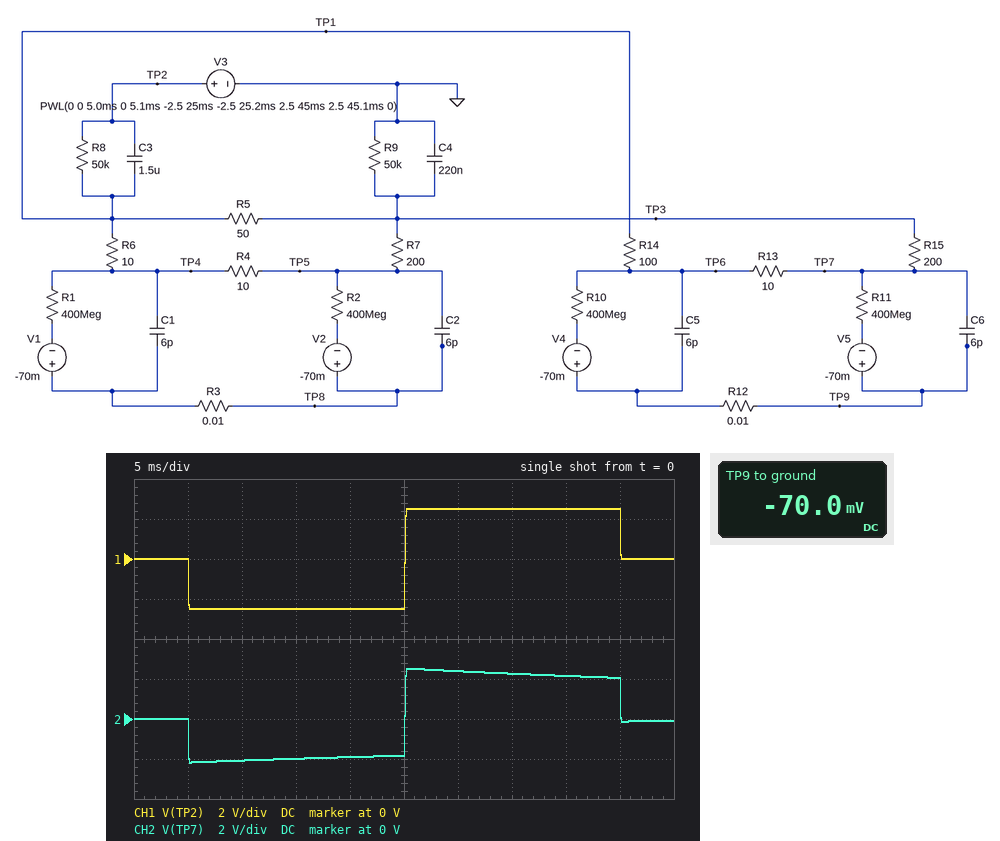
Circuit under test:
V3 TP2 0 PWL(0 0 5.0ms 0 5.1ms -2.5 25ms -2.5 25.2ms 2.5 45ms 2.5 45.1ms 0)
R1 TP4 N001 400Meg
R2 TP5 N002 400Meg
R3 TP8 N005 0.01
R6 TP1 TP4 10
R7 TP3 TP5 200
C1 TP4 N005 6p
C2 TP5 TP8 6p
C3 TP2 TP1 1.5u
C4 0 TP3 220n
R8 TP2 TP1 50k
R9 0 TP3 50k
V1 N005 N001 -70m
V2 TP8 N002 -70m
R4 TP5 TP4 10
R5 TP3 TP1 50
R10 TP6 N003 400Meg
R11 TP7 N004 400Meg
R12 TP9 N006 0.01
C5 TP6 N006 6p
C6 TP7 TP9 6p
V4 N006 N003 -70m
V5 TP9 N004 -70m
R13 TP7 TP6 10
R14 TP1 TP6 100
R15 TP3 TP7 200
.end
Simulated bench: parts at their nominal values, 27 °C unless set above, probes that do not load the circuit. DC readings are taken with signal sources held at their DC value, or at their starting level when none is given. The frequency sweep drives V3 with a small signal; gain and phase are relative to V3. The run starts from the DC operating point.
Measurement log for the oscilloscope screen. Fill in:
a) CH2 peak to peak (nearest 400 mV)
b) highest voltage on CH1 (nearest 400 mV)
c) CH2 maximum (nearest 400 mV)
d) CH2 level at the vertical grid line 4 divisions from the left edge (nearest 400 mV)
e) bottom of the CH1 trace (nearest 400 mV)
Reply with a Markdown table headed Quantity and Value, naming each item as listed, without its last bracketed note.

| Quantity | Value |
|---|---|
| CH2 peak to peak | 4.8 V |
| highest voltage on CH1 | 2.4 V |
| CH2 maximum | 2.4 V |
| CH2 level at the vertical grid line 4 divisions from the left edge | -2.0 V |
| bottom of the CH1 trace | -2.4 V |
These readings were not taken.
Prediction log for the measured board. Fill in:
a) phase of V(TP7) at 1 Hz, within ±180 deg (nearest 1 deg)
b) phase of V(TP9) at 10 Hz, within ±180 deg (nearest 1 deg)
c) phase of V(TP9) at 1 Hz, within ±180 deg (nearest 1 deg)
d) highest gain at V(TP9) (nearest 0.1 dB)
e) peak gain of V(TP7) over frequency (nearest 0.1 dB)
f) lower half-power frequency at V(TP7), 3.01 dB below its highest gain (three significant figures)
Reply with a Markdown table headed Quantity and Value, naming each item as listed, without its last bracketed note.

| Quantity | Value |
|---|---|
| phase of V(TP7) at 1 Hz, within ±180 deg | 10 deg |
| phase of V(TP9) at 10 Hz, within ±180 deg | 8 deg |
| phase of V(TP9) at 1 Hz, within ±180 deg | 10 deg |
| highest gain at V(TP9) | -1.2 dB |
| peak gain of V(TP7) over frequency | -1.2 dB |
| lower half-power frequency at V(TP7), 3.01 dB below its highest gain | 2.16 Hz |
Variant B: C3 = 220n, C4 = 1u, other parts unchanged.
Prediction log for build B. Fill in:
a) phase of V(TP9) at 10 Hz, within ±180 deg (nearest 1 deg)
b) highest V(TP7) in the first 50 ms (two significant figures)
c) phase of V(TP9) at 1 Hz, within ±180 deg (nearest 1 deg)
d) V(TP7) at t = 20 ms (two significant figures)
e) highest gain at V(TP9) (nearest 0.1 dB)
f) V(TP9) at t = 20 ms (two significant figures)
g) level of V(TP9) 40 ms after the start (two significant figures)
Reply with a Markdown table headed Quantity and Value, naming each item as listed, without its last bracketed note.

| Quantity | Value |
|---|---|
| phase of V(TP9) at 10 Hz, within ±180 deg | -28 deg |
| highest V(TP7) in the first 50 ms | 630 mV |
| phase of V(TP9) at 1 Hz, within ±180 deg | -7 deg |
| V(TP7) at t = 20 ms | -760 mV |
| highest gain at V(TP9) | -6.0 dB |
| V(TP9) at t = 20 ms | -830 mV |
| level of V(TP9) 40 ms after the start | 450 mV |
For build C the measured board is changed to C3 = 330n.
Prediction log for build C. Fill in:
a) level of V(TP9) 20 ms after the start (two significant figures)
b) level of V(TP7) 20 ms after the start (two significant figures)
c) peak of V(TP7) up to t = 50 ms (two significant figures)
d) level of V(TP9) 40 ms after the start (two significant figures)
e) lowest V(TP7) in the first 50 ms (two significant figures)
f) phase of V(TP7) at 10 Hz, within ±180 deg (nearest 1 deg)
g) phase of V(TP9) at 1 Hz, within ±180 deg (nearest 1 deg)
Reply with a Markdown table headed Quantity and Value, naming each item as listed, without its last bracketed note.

| Quantity | Value |
|---|---|
| level of V(TP9) 20 ms after the start | -1.4 V |
| level of V(TP7) 20 ms after the start | -1.3 V |
| peak of V(TP7) up to t = 50 ms | 1.7 V |
| level of V(TP9) 40 ms after the start | 1.3 V |
| lowest V(TP7) in the first 50 ms | -1.5 V |
| phase of V(TP7) at 10 Hz, within ±180 deg | 5 deg |
| phase of V(TP9) at 1 Hz, within ±180 deg | 1 deg |
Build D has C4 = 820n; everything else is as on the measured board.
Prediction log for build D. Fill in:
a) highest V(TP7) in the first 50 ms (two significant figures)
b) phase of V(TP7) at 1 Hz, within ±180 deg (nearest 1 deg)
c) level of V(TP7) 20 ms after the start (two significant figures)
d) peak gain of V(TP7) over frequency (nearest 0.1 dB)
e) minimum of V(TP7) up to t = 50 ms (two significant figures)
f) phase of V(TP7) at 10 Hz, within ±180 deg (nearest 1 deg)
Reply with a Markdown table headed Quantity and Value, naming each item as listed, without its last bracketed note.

| Quantity | Value |
|---|---|
| highest V(TP7) in the first 50 ms | 1.7 V |
| phase of V(TP7) at 1 Hz, within ±180 deg | 5 deg |
| level of V(TP7) 20 ms after the start | -1.5 V |
| peak gain of V(TP7) over frequency | -3.8 dB |
| minimum of V(TP7) up to t = 50 ms | -1.6 V |
| phase of V(TP7) at 10 Hz, within ±180 deg | 3 deg |
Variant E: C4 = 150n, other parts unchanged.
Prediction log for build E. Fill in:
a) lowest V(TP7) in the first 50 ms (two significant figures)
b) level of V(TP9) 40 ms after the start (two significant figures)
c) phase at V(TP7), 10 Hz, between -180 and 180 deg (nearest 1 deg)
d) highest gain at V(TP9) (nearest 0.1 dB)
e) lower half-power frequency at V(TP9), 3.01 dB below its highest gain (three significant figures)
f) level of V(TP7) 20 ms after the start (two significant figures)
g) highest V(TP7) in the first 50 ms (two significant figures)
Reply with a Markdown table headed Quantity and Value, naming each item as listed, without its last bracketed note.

| Quantity | Value |
|---|---|
| lowest V(TP7) in the first 50 ms | -2.3 V |
| level of V(TP9) 40 ms after the start | 2.2 V |
| phase at V(TP7), 10 Hz, between -180 and 180 deg | 9 deg |
| highest gain at V(TP9) | -0.8 dB |
| lower half-power frequency at V(TP9), 3.01 dB below its highest gain | 2.42 Hz |
| level of V(TP7) 20 ms after the start | -2.0 V |
| highest V(TP7) in the first 50 ms | 2.7 V |
